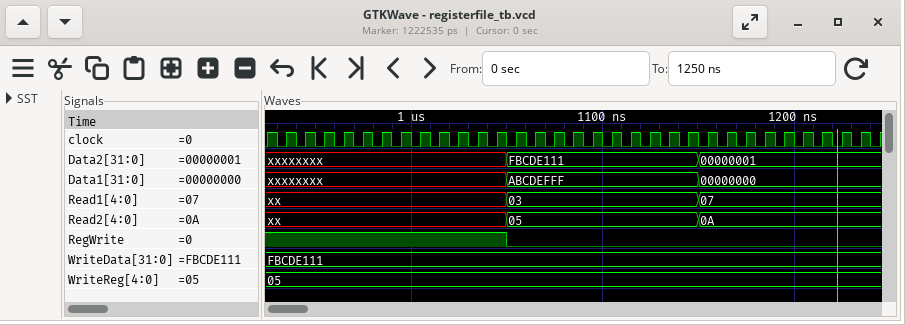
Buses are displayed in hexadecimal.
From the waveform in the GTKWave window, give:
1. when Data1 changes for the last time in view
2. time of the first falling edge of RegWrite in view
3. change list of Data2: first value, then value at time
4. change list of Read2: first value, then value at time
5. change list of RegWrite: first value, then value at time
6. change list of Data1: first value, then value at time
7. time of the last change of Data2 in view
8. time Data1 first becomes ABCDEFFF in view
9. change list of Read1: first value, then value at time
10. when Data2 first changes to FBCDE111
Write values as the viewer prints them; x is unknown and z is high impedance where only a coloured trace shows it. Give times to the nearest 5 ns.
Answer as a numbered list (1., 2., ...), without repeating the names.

1. 1150 ns
2. 1050 ns
3. xxxxxxxx, FBCDE111 at 1050 ns, 00000001 at 1150 ns
4. xx, 05 at 1050 ns, 0A at 1150 ns
5. 1, 0 at 1050 ns
6. xxxxxxxx, ABCDEFFF at 1050 ns, 00000000 at 1150 ns
7. 1150 ns
8. 1050 ns
9. xx, 03 at 1050 ns, 07 at 1150 ns
10. 1050 ns
